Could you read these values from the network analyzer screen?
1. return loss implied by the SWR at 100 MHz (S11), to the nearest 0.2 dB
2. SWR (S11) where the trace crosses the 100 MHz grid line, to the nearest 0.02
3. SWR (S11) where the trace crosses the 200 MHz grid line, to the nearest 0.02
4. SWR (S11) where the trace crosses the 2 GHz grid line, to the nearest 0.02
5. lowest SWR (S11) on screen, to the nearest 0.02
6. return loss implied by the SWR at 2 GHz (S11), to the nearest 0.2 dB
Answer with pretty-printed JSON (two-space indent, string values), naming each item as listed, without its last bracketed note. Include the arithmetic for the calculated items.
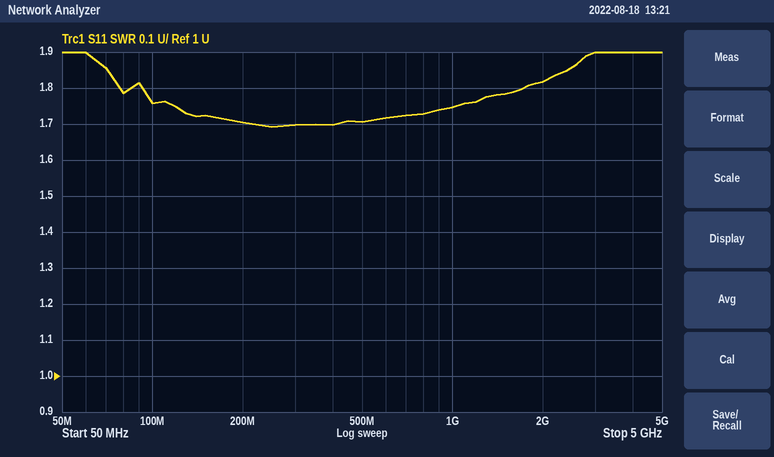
{
  "return loss implied by the SWR at 100 MHz (S11), to the nearest 0.2 dB": "−20 log10((1.76 − 1)/(1.76 + 1)) ≈ 11.2 dB",
  "SWR (S11) where the trace crosses the 100 MHz grid line, to the nearest 0.02": "1.76",
  "SWR (S11) where the trace crosses the 200 MHz grid line, to the nearest 0.02": "1.70",
  "SWR (S11) where the trace crosses the 2 GHz grid line, to the nearest 0.02": "1.82",
  "lowest SWR (S11) on screen, to the nearest 0.02": "1.70",
  "return loss implied by the SWR at 2 GHz (S11), to the nearest 0.2 dB": "−20 log10((1.82 − 1)/(1.82 + 1)) ≈ 10.7 dB, so 10.8 dB to the nearest 0.2 dB"
}
